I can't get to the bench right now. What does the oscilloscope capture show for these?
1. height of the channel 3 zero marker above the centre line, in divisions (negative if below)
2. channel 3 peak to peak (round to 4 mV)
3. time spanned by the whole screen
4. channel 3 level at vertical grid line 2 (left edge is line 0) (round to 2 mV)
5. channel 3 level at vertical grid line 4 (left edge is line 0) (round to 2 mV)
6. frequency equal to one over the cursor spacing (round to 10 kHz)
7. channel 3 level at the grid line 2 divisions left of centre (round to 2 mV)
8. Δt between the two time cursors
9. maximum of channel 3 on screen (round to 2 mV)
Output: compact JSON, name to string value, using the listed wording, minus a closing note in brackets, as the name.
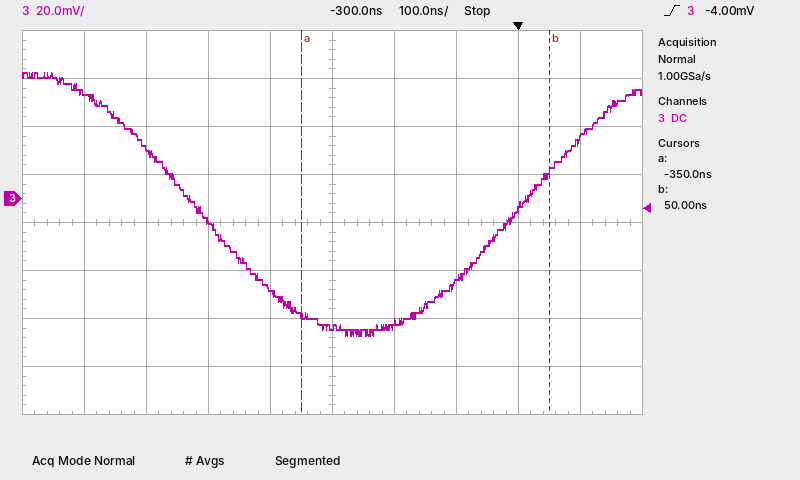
{"height of the channel 3 zero marker above the centre line, in divisions": "+0.5 div", "channel 3 peak to peak": "108 mV", "time spanned by the whole screen": "1 µs", "channel 3 level at vertical grid line 2 (left edge is line 0)": "20 mV", "channel 3 level at vertical grid line 4 (left edge is line 0)": "-38 mV", "frequency equal to one over the cursor spacing": "2.50 MHz", "channel 3 level at the grid line 2 divisions left of centre": "-10 mV", "Δt between the two time cursors": "400 ns", "maximum of channel 3 on screen": "52 mV"}
